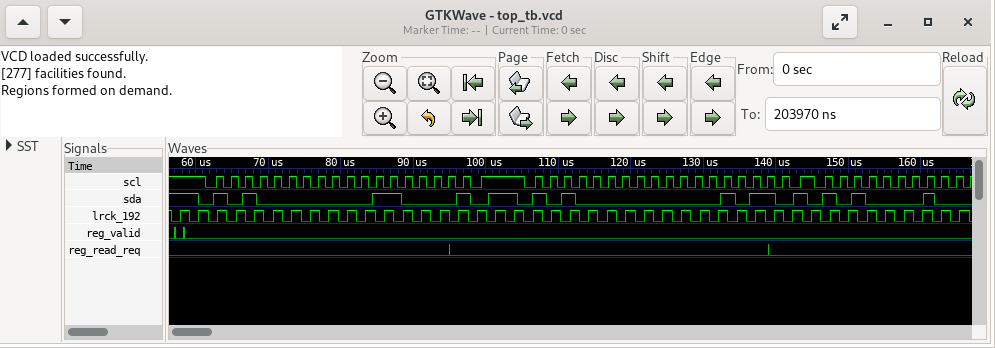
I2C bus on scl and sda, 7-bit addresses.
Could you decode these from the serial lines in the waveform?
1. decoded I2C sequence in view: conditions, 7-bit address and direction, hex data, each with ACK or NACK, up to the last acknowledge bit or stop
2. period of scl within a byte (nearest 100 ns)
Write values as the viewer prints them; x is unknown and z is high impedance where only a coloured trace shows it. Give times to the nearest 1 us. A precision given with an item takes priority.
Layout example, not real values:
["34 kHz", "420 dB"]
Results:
["start, address 50 write ACK, 30 NACK, stop, start, address 50 write ACK, 0B ACK, repeated start, address 50 read ACK", "2000 ns"]
